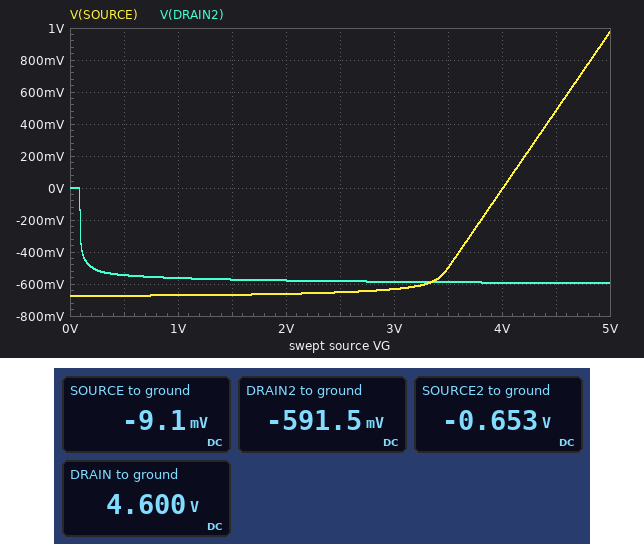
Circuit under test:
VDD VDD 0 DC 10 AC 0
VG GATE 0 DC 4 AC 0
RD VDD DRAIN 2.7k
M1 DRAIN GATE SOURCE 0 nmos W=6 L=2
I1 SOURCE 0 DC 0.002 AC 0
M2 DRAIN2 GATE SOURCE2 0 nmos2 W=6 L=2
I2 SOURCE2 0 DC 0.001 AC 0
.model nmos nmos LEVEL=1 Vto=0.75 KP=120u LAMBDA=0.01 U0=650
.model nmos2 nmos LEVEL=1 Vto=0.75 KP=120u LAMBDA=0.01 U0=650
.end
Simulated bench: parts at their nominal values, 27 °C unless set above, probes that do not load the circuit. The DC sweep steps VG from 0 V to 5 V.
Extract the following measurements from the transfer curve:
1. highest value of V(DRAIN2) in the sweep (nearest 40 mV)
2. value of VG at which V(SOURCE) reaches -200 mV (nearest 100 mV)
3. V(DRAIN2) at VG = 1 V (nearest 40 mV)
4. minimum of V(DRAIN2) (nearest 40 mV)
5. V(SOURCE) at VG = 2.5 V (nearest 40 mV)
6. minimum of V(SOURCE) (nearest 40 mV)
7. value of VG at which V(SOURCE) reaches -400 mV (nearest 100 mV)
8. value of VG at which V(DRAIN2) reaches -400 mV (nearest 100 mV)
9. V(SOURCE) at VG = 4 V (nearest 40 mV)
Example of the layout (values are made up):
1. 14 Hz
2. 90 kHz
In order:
1. 0 V
2. 3.8 V
3. -560 mV
4. -600 mV
5. -640 mV
6. -680 mV
7. 3.6 V
8. 100 mV
9. 0 V
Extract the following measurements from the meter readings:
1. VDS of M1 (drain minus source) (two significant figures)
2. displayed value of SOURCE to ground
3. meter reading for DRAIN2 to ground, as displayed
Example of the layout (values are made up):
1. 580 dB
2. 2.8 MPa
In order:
1. 4.6 V
2. -9.1 mV
3. -591.5 mV
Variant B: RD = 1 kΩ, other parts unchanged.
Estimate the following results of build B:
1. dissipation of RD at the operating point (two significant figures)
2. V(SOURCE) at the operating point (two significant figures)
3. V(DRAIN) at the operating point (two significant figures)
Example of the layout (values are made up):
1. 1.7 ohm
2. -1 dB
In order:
1. 4.0 mW
2. 42 mV
3. 8.0 V
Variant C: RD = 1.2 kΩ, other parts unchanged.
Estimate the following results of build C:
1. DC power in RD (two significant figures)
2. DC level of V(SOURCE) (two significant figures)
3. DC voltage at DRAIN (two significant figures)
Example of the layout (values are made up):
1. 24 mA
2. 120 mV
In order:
1. 4.8 mW
2. 36 mV
3. 7.6 V
